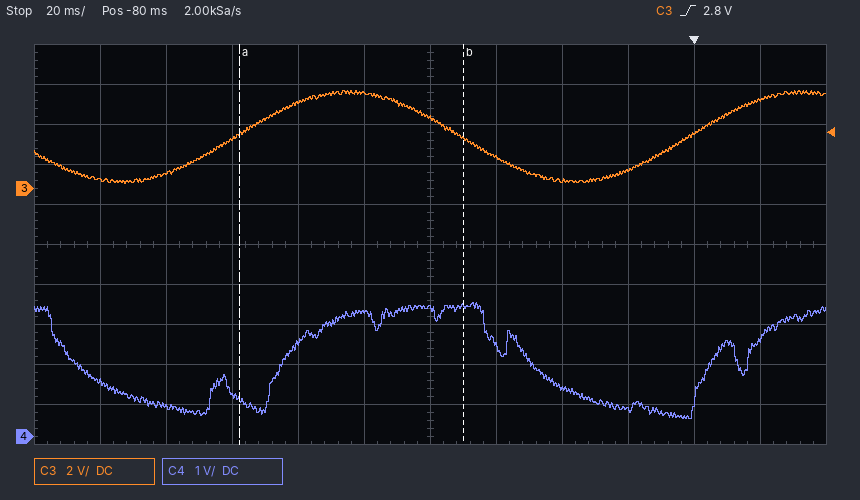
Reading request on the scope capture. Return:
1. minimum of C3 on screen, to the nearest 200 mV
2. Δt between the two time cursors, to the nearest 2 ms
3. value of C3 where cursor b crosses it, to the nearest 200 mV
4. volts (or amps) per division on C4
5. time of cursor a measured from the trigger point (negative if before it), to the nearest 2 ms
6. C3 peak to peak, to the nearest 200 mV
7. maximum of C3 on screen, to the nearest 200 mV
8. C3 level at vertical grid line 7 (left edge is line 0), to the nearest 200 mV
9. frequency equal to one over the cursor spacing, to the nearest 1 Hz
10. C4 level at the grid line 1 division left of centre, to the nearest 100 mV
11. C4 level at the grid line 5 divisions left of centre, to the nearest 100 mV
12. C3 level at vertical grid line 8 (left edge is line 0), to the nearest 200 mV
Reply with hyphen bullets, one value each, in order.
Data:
- 200 mV
- 68 ms
- 2.6 V
- 1 V
- -138 ms
- 4.6 V
- 4.8 V
- 1.6 V
- 15 Hz
- 3.1 V
- 1.4 V
- 400 mV
